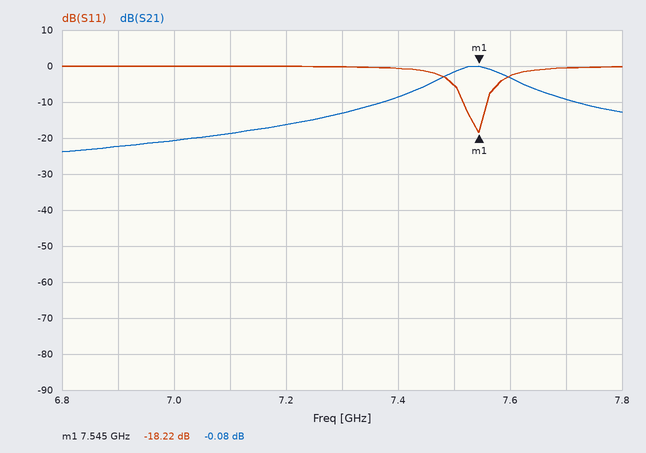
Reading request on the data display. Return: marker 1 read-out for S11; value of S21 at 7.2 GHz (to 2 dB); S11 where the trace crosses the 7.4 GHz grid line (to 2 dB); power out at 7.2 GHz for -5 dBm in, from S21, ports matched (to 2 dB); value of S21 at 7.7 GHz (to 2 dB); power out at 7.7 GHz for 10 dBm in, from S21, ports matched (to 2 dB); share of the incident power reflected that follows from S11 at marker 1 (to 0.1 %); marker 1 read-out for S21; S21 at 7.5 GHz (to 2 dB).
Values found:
-18.22 dB
-16 dB
0 dB
-22 dBm
-10 dB
0 dBm
1.5 %
-0.08 dB
-2 dB
